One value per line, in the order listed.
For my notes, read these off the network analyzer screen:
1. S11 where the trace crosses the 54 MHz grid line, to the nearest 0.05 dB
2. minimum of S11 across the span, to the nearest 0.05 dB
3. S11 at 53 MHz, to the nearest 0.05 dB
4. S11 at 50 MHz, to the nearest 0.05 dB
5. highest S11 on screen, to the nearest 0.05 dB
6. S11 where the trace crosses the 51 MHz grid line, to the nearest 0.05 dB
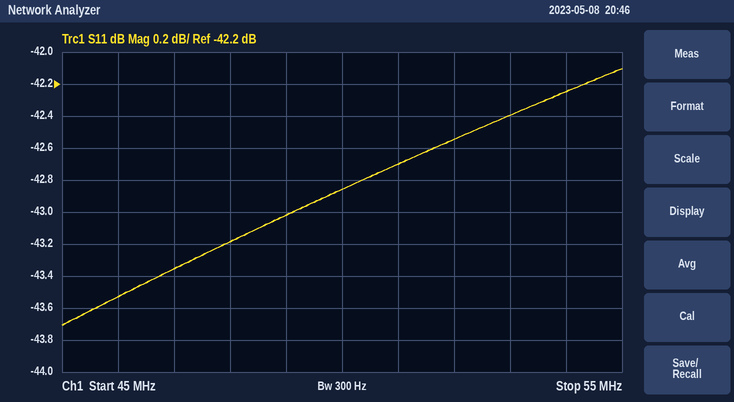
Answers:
-42.25 dB
-43.70 dB
-42.40 dB
-42.85 dB
-42.10 dB
-42.70 dB
